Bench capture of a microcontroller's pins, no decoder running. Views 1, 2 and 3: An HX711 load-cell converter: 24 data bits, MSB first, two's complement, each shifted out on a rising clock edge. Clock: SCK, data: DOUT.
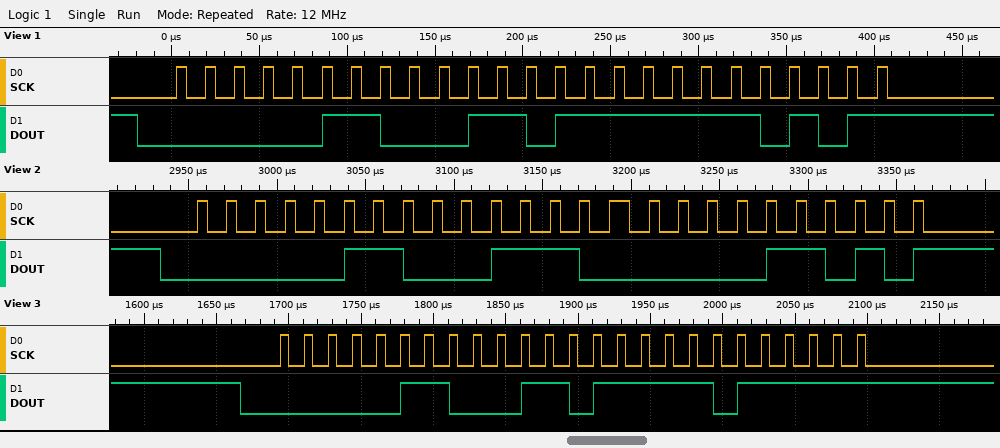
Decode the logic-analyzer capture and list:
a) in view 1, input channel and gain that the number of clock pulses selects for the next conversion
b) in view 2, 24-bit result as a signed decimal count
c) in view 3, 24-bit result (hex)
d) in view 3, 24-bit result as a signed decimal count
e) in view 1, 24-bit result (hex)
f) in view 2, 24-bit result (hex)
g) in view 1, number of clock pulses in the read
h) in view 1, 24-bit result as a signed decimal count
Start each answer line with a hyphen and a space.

- channel A, gain 128
- 407578
- 0x0637DF
- 407519
- 0x0637F5
- 0x06381A
- 25
- 407541
